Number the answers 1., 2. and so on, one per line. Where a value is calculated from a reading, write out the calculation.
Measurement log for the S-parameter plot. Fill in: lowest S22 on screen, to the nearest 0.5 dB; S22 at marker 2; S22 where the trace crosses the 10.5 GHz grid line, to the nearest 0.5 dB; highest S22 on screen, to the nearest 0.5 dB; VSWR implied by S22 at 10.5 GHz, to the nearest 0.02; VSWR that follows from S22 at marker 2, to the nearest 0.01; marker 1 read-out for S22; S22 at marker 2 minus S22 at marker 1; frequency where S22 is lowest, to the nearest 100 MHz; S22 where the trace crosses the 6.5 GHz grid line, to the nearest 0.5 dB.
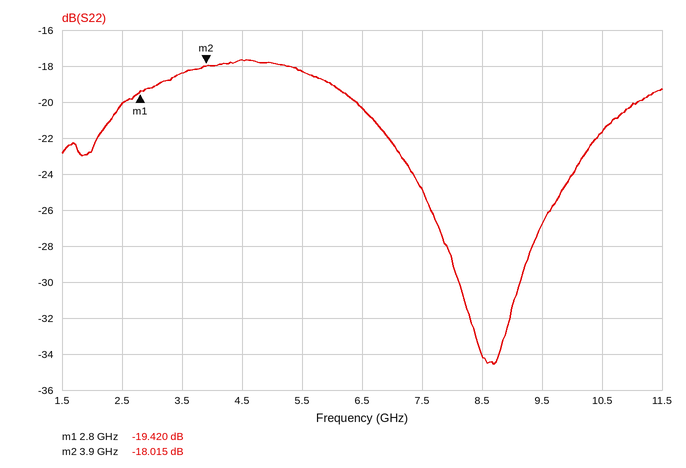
1. -34.5 dB
2. -18.015 dB
3. -21.5 dB
4. -17.5 dB
5. |Γ| = 10^(-21.5/20) = 0.0841; VSWR = (1 + 0.0841)/(1 − 0.0841) ≈ 1.18
6. (1 + 0.1257)/(1 − 0.1257) ≈ 1.29
7. -19.420 dB
8. -18.015 − (-19.42) = 1.405 dB
9. 8.7 GHz
10. -20.5 dB
